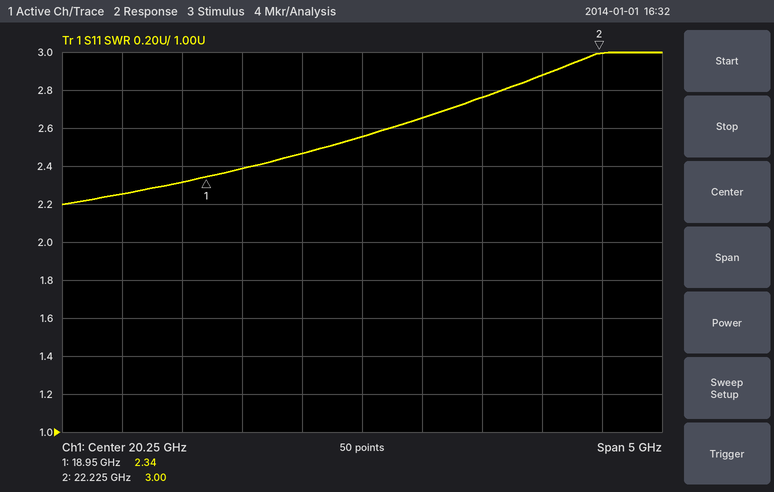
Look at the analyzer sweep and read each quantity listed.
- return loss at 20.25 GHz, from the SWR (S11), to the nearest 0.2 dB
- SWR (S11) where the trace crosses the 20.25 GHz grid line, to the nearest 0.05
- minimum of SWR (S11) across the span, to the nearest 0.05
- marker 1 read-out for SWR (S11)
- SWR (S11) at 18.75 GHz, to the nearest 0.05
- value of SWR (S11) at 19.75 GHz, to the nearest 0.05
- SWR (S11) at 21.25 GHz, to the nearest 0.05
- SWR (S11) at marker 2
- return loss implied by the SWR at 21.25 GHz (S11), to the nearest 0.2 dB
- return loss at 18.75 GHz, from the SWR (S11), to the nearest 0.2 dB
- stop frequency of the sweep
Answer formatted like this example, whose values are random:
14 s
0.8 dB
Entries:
7.2 dB
2.55
2.20
2.34
2.30
2.45
2.75
3.00
6.6 dB
8.0 dB
22.75 GHz
